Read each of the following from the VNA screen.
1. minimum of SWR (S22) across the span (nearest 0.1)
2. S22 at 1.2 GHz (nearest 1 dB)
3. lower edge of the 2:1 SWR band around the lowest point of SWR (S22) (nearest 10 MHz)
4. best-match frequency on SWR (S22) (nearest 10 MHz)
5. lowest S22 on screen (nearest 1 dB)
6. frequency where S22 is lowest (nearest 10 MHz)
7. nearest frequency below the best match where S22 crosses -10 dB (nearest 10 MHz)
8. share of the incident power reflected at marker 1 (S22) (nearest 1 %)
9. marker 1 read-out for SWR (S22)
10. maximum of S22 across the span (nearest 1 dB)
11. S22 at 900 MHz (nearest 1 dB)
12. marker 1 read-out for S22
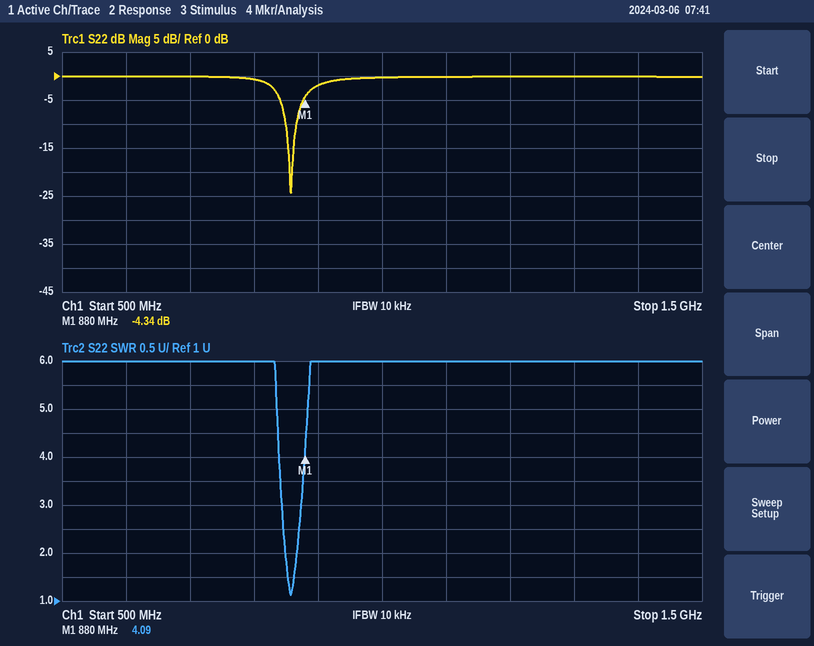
1.1
0 dB
850 MHz
860 MHz
-24 dB
860 MHz
850 MHz
37 %
4.09
0 dB
-2 dB
-4.34 dB
